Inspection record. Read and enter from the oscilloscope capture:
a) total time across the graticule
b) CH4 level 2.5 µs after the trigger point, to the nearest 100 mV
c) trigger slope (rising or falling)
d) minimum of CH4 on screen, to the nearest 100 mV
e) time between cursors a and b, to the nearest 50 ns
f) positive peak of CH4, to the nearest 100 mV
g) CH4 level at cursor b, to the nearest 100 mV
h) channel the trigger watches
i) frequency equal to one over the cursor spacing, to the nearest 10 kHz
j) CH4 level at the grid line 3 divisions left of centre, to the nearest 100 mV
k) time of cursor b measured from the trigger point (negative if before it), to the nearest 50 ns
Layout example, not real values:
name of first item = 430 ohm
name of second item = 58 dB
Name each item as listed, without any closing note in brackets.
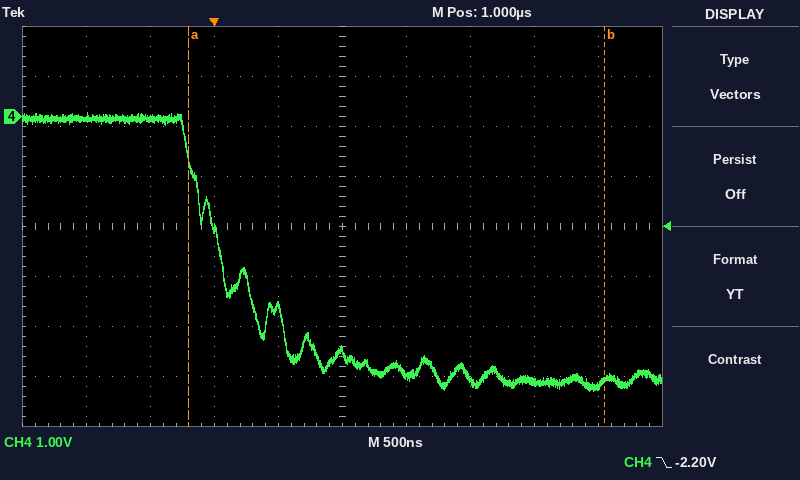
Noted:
total time across the graticule = 5 µs
CH4 level 2.5 µs after the trigger point, to the nearest 100 mV = -5.3 V
trigger slope = falling
minimum of CH4 on screen, to the nearest 100 mV = -5.5 V
time between cursors a and b, to the nearest 50 ns = 3.25 µs
positive peak of CH4, to the nearest 100 mV = 100 mV
CH4 level at cursor b, to the nearest 100 mV = -5.3 V
channel the trigger watches = CH4
frequency equal to one over the cursor spacing, to the nearest 10 kHz = 310 kHz
CH4 level at the grid line 3 divisions left of centre, to the nearest 100 mV = 0.0 V
time of cursor b measured from the trigger point (negative if before it), to the nearest 50 ns = +3.05 µs
